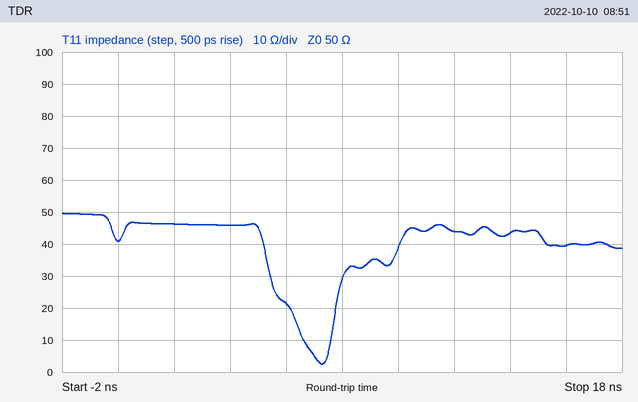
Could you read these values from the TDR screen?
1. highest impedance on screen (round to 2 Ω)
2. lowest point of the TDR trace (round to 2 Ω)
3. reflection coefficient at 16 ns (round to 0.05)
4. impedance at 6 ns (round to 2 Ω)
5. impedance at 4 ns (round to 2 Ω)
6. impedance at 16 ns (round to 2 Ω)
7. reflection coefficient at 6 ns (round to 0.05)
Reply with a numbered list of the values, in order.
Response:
1. 50 Ω
2. 2 Ω
3. -0.10
4. 22 Ω
5. 46 Ω
6. 40 Ω
7. -0.40
